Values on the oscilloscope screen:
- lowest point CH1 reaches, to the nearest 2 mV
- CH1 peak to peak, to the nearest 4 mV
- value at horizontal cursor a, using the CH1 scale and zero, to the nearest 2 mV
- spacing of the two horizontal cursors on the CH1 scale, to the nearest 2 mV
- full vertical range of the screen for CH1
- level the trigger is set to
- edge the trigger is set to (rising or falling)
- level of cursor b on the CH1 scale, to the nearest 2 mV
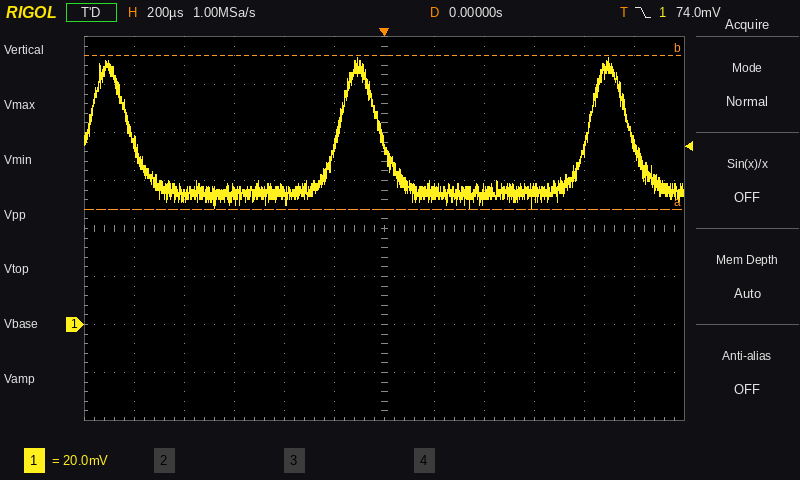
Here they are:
48 mV
64 mV
48 mV
64 mV
160 mV
74.0 mV
falling
112 mV
